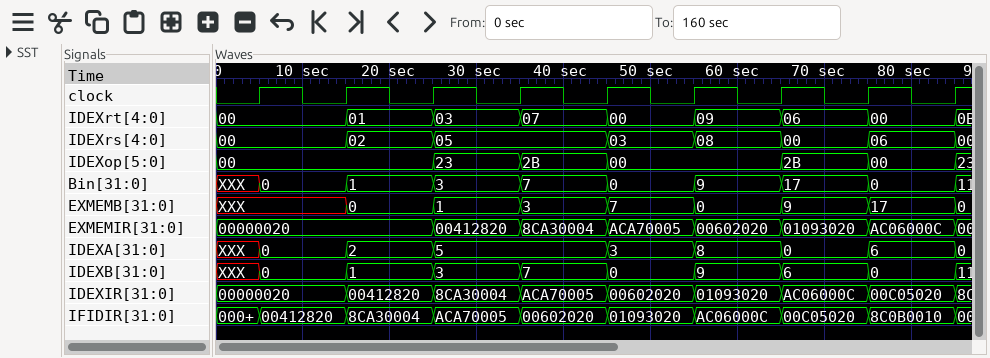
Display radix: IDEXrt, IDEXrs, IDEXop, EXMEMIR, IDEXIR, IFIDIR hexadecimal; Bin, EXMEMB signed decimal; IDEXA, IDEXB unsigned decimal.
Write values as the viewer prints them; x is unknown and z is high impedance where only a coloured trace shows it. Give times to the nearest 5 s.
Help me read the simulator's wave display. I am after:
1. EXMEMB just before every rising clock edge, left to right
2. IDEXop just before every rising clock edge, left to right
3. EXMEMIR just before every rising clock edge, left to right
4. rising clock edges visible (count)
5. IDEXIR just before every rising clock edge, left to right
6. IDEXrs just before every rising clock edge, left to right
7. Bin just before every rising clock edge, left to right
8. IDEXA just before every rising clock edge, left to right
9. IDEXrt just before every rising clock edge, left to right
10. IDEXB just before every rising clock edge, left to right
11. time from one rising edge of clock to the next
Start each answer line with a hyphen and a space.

- XXX, XXX, 0, 1, 3, 7, 0, 9, 17
- 00, 00, 00, 23, 2B, 00, 00, 2B, 00
- 00000020, 00000020, 00000020, 00412820, 8CA30004, ACA70005, 00602020, 01093020, AC06000C
- 9
- 00000020, 00000020, 00412820, 8CA30004, ACA70005, 00602020, 01093020, AC06000C, 00C05020
- 00, 00, 02, 05, 05, 03, 08, 00, 06
- XXX, 0, 1, 3, 7, 0, 9, 17, 0
- XXX, 0, 2, 5, 5, 3, 8, 0, 6
- 00, 00, 01, 03, 07, 00, 09, 06, 00
- XXX, 0, 1, 3, 7, 0, 9, 6, 0
- 10 s
